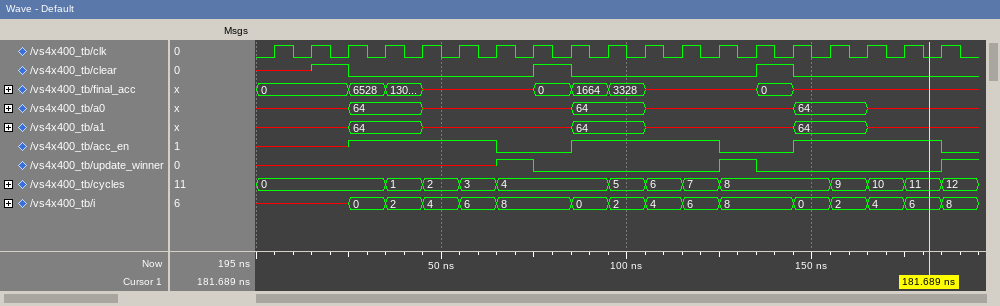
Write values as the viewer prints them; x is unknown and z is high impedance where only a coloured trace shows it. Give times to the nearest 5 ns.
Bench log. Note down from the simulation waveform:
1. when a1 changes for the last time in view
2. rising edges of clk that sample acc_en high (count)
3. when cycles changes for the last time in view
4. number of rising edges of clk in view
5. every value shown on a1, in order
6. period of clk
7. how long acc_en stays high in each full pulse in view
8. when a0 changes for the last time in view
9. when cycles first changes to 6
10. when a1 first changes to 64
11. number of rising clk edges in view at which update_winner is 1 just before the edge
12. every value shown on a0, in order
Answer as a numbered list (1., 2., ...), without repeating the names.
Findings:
1. 165 ns
2. 12
3. 185 ns
4. 19
5. x, 64, x, 64, x, 64, x
6. 10 ns
7. 40 ns, 40 ns
8. 165 ns
9. 105 ns
10. 25 ns
11. 2
12. x, 64, x, 64, x, 64, x
